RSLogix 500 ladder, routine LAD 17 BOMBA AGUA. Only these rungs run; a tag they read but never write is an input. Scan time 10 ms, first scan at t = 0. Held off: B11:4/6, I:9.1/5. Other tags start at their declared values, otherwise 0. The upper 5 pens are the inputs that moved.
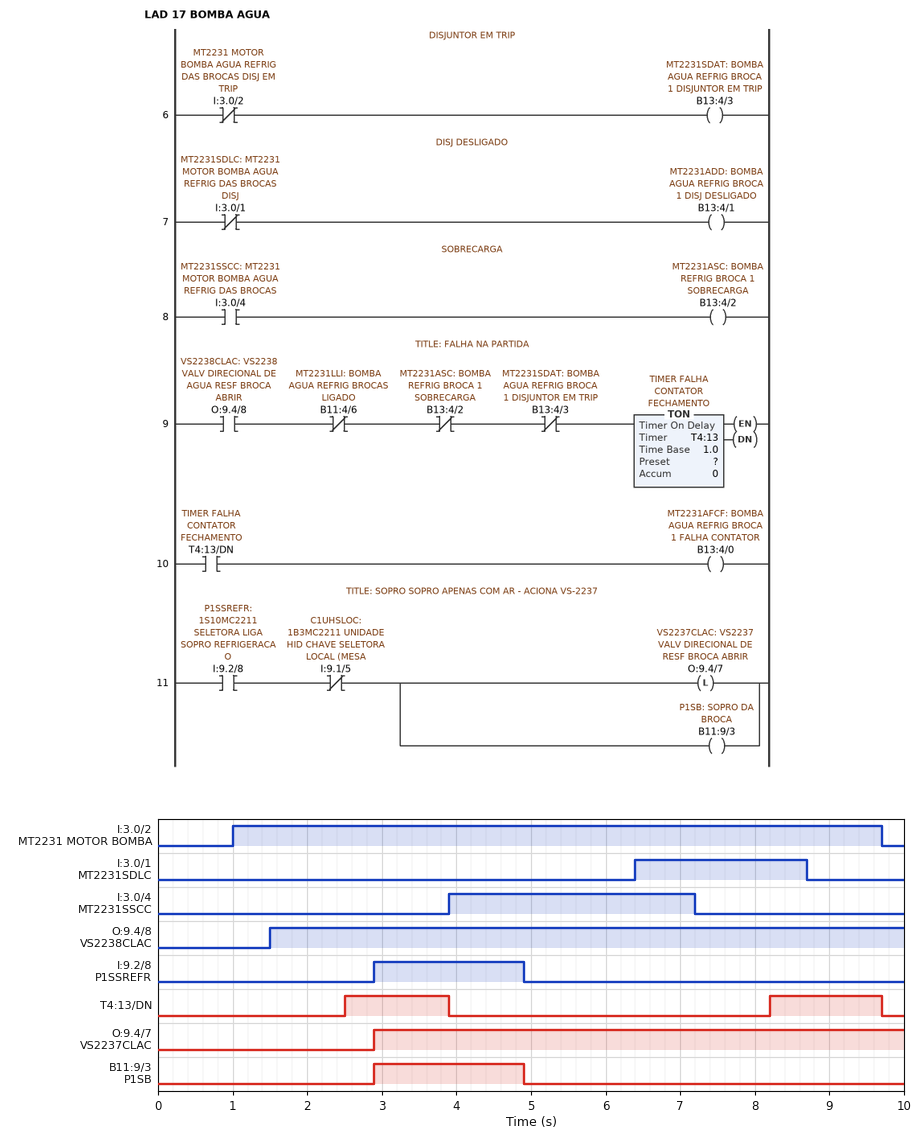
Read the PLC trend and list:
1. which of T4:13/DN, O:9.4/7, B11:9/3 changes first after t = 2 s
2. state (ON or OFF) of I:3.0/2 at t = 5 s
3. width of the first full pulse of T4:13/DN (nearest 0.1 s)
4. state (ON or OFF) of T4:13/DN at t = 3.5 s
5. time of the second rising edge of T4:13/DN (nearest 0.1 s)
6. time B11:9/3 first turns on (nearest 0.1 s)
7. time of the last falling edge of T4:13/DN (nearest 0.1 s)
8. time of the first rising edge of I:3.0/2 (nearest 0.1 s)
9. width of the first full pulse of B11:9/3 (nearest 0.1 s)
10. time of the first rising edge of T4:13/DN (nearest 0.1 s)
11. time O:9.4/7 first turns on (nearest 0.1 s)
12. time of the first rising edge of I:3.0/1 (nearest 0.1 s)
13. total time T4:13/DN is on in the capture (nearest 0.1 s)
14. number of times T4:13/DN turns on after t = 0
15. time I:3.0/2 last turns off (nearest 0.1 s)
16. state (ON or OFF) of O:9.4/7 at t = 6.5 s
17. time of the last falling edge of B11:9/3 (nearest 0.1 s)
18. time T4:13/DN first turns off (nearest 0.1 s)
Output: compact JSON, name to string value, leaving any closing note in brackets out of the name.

{"which of T4:13/DN, O:9.4/7, B11:9/3 changes first after t = 2 s": "T4:13/DN", "state (ON or OFF) of I:3.0/2 at t = 5 s": "ON", "width of the first full pulse of T4:13/DN": "1.4 s", "state (ON or OFF) of T4:13/DN at t = 3.5 s": "ON", "time of the second rising edge of T4:13/DN": "8.2 s", "time B11:9/3 first turns on": "2.9 s", "time of the last falling edge of T4:13/DN": "9.7 s", "time of the first rising edge of I:3.0/2": "1.0 s", "width of the first full pulse of B11:9/3": "2.0 s", "time of the first rising edge of T4:13/DN": "2.5 s", "time O:9.4/7 first turns on": "2.9 s", "time of the first rising edge of I:3.0/1": "6.4 s", "total time T4:13/DN is on in the capture": "2.9 s", "number of times T4:13/DN turns on after t = 0": "2", "time I:3.0/2 last turns off": "9.7 s", "state (ON or OFF) of O:9.4/7 at t = 6.5 s": "ON", "time of the last falling edge of B11:9/3": "4.9 s", "time T4:13/DN first turns off": "3.9 s"}
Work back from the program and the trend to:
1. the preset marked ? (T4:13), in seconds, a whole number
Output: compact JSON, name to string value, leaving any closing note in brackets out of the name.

{"the preset marked ? (T4:13), in seconds, a whole number": "1 s"}
